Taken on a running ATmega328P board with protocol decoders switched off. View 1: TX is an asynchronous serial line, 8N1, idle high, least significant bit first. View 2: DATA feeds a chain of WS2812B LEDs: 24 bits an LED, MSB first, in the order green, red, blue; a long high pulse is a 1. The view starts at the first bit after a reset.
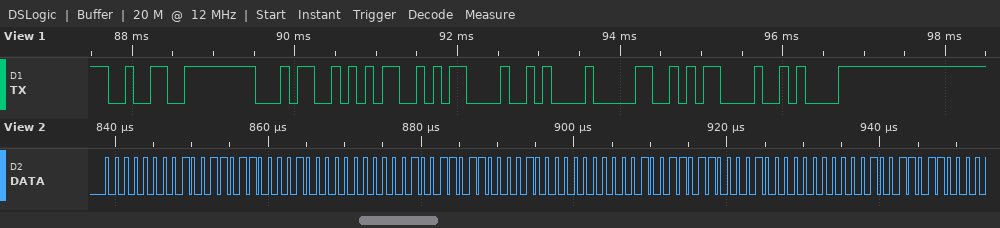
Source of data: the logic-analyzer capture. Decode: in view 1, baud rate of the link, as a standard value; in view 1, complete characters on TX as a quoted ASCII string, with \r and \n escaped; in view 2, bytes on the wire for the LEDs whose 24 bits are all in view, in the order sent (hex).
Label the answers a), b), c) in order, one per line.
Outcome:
a) 9600 baud
b) "245\r\n0\r\n"
c) 00 9B 08 00 9B 08 00 9B 08
